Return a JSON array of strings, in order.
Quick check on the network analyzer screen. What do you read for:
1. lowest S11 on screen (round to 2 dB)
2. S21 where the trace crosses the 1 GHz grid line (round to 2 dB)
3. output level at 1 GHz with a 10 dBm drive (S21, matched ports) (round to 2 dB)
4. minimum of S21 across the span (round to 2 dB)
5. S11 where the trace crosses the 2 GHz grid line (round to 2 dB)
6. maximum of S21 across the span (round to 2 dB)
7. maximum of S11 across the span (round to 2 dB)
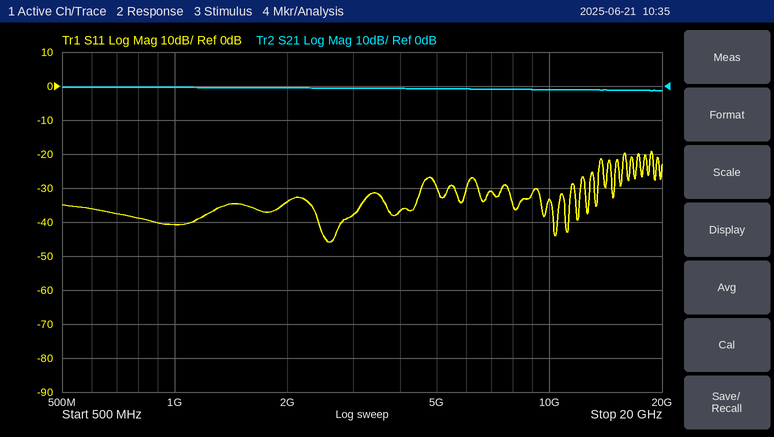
["-46 dB", "0 dB", "10 dBm", "-2 dB", "-34 dB", "0 dB", "-20 dB"]
